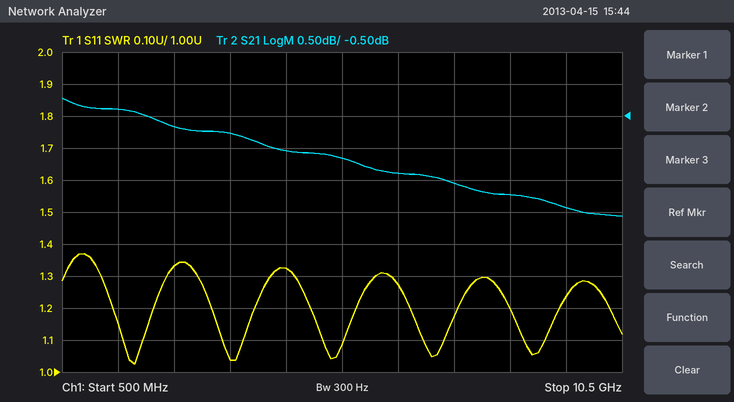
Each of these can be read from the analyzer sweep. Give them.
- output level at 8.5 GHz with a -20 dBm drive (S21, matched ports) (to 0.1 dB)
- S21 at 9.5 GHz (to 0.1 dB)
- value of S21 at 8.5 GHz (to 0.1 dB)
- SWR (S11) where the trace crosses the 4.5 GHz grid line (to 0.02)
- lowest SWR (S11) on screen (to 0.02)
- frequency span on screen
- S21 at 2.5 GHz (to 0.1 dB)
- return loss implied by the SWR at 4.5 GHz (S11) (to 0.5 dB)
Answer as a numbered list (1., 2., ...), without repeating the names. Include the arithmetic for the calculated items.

1. -20 dBm + (-1.7 dB) = -21.7 dBm
2. -1.9 dB
3. -1.7 dB
4. 1.32
5. 1.02
6. 10 GHz
7. -0.7 dB
8. −20 log10((1.32 − 1)/(1.32 + 1)) ≈ 17.2 dB, so 17.0 dB to the nearest 0.5 dB
